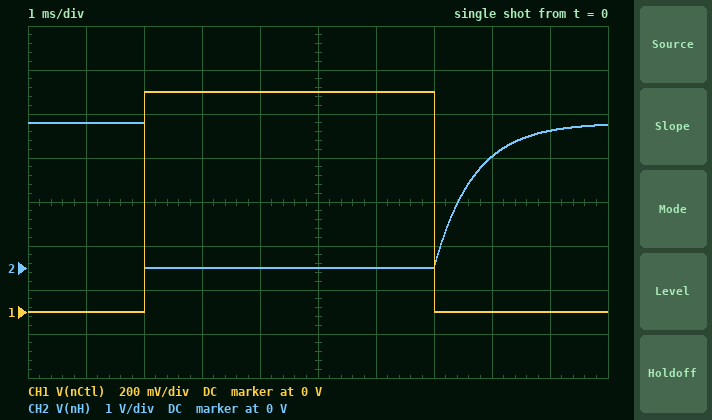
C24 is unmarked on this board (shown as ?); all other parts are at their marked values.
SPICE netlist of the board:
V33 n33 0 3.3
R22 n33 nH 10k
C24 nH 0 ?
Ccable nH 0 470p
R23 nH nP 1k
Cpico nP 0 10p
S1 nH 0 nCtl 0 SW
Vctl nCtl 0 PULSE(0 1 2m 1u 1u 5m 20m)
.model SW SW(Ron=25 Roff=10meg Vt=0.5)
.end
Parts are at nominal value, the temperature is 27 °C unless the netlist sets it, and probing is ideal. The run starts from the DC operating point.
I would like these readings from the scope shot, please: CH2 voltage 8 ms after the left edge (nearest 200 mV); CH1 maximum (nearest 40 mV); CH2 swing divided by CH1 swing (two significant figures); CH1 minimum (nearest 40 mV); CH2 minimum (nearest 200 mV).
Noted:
2.6 V
1.00 V
3.3
0 V
0 V
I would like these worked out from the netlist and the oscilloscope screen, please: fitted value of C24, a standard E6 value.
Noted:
68 nF
